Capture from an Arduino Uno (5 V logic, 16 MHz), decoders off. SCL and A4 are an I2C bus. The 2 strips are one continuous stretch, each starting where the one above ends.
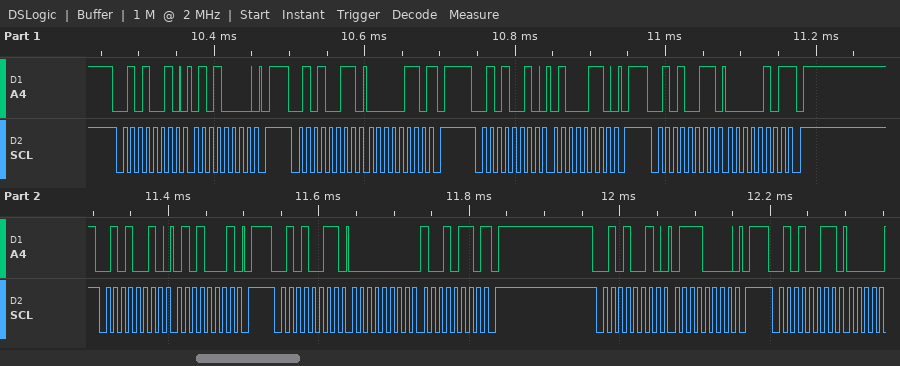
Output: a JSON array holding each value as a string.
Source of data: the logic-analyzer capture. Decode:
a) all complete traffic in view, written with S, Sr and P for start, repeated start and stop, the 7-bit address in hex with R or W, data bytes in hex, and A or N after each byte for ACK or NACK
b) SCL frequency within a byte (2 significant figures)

["S 29W A 50 A P S 29R A 06 N P S 29W A 46 A P S 29R A 05 N P S 29W A 51 A P S 29R A 00 A 96 N P S 29W A 70 A P S 29R A", "100 kHz"]
